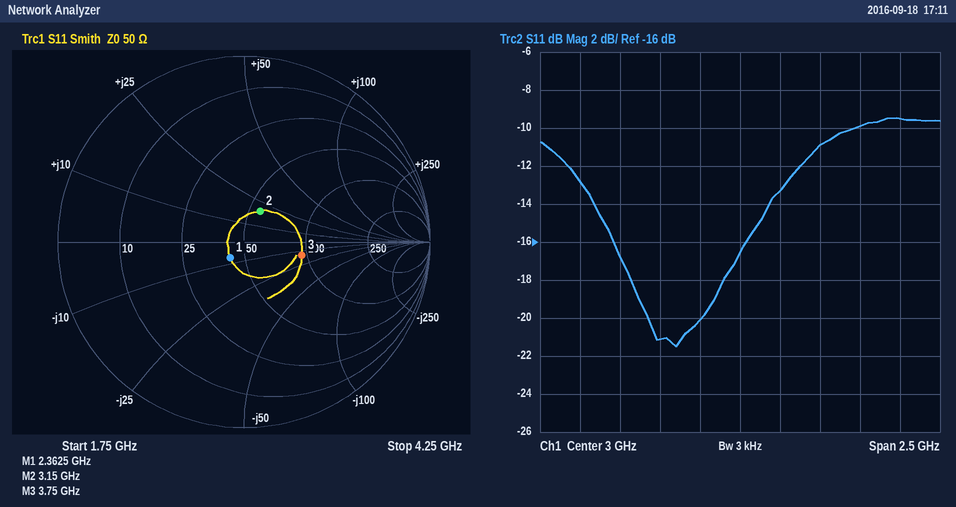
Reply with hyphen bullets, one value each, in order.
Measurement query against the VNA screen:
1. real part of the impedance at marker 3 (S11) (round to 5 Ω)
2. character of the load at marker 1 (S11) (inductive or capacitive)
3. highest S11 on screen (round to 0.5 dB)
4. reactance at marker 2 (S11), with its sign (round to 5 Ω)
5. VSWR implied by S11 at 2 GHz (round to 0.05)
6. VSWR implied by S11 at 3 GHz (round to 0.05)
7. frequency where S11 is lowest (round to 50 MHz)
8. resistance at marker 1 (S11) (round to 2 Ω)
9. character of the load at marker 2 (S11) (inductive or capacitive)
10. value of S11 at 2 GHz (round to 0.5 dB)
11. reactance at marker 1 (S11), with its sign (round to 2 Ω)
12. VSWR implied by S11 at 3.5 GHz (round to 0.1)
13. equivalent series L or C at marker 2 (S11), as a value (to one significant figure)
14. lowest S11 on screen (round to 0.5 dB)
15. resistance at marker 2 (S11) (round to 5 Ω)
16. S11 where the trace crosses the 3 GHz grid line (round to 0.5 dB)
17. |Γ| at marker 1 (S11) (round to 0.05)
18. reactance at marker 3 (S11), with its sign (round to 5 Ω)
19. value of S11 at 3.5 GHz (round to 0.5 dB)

- 95 Ω
- capacitive
- -9.5 dB
- +20 Ω
- 1.60
- 1.35
- 2.60 GHz
- 42 Ω
- inductive
- -13.0 dB
- -8 Ω
- 1.8
- 1.0 nH
- -21.5 dB
- 55 Ω
- -16.5 dB
- 0.10
- -15 Ω
- -11.0 dB
